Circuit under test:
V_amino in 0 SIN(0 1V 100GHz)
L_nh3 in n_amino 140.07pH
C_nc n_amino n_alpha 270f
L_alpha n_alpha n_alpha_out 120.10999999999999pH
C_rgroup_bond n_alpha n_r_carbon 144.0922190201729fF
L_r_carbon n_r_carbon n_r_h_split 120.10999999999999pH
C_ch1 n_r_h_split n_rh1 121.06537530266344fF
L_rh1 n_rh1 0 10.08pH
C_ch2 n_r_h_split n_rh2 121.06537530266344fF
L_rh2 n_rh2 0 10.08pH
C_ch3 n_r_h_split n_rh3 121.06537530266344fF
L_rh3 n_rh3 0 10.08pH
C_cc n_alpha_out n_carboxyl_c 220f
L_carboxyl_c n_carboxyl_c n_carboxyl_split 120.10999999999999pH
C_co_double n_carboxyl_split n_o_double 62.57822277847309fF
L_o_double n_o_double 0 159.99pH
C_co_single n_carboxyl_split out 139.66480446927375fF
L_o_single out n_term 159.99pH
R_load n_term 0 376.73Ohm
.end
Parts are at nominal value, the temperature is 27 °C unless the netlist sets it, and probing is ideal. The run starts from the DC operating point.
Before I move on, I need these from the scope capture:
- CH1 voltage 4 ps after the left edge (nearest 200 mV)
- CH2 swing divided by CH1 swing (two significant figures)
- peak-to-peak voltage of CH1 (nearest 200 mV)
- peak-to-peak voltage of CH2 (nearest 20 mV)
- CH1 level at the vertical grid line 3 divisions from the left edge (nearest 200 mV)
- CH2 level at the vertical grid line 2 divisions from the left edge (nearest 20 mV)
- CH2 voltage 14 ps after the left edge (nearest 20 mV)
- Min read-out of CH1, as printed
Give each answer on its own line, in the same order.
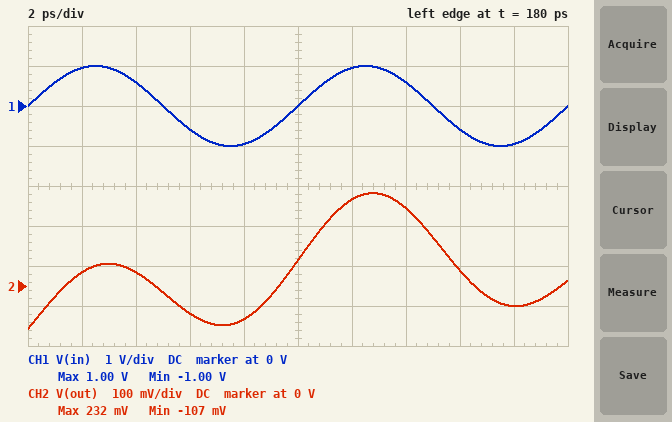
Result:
600 mV
0.17
2.0 V
340 mV
-600 mV
40 mV
200 mV
-1.00 V
